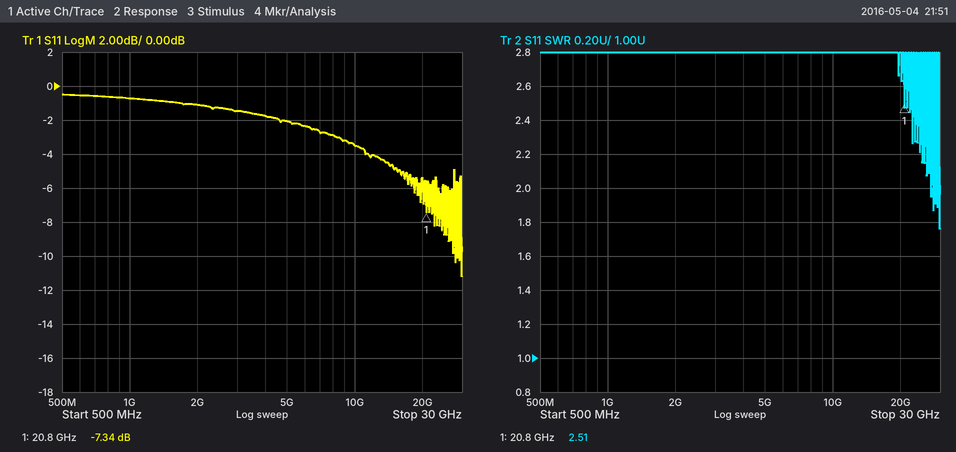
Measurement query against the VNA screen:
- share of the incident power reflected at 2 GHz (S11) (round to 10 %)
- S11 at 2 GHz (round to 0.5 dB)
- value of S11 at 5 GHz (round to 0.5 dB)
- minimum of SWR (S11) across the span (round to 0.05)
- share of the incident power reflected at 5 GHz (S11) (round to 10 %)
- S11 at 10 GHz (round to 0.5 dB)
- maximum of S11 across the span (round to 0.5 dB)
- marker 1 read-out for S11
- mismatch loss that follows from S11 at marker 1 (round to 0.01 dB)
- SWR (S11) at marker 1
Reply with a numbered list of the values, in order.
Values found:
1. 80 %
2. -1.0 dB
3. -2.0 dB
4. 1.75
5. 60 %
6. -3.5 dB
7. -0.5 dB
8. -7.34 dB
9. 0.89 dB
10. 2.51
